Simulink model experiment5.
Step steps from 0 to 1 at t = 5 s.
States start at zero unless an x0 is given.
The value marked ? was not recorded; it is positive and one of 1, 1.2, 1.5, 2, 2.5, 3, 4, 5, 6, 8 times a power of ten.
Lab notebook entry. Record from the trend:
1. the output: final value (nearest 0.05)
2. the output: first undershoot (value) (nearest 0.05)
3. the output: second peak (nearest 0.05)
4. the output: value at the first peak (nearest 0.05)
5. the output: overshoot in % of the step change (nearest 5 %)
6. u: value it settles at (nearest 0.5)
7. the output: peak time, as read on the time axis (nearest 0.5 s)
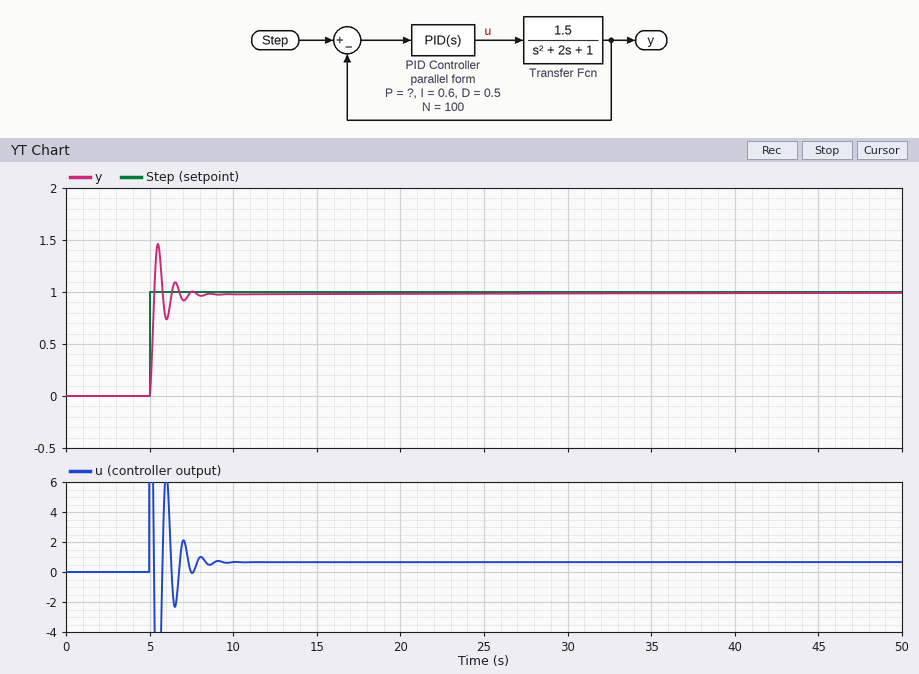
1.00
0.75
1.10
1.45
45 %
0.5
5.5 s
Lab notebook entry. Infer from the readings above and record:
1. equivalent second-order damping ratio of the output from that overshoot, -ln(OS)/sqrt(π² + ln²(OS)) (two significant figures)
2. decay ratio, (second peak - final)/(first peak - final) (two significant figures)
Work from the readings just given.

0.25
0.22
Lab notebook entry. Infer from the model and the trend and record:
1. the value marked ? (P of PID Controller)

25
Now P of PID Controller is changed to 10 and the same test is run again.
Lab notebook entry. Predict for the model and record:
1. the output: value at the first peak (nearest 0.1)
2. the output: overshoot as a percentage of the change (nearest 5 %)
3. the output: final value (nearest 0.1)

1.3
25 %
1.0
